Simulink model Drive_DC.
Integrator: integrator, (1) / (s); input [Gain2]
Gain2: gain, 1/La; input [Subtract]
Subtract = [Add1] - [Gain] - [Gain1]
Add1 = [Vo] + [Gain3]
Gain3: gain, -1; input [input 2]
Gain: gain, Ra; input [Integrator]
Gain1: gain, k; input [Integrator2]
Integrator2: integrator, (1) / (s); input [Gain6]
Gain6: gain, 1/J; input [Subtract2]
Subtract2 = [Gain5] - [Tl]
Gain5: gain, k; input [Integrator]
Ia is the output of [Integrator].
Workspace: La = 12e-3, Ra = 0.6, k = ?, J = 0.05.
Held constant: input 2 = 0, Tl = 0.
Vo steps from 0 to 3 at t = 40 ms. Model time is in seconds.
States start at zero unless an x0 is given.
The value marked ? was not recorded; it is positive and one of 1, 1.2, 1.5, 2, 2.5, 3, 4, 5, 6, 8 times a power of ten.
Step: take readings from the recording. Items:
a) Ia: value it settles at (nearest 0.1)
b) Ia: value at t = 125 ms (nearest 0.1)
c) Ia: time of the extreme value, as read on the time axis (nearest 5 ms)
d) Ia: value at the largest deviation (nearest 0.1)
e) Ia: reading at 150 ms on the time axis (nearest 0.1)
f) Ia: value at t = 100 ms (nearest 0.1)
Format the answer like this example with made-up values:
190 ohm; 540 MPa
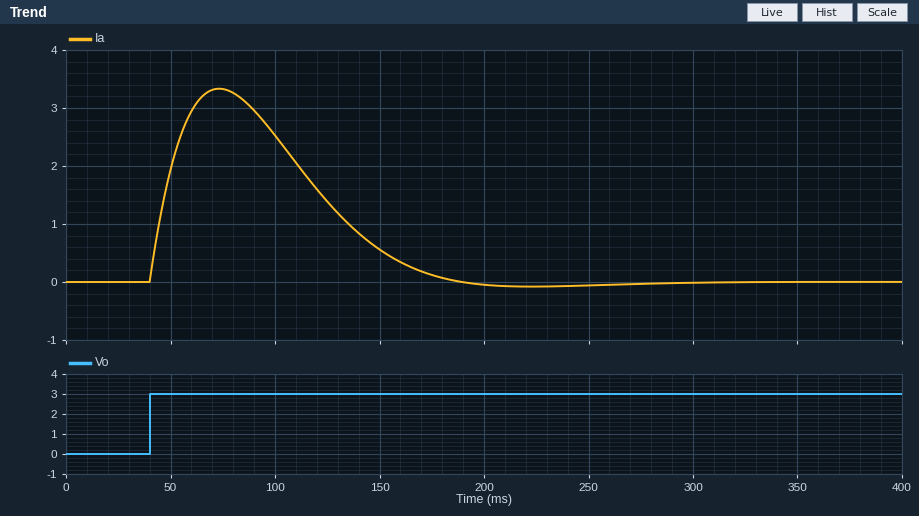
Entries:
0.0; 1.4; 75 ms; 3.3; 0.6; 2.5
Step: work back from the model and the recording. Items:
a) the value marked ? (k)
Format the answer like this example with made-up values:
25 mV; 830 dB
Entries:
0.8
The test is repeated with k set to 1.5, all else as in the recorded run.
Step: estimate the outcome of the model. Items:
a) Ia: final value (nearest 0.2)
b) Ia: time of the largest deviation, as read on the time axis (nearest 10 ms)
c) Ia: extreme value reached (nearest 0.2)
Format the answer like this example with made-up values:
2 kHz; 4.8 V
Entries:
0.0; 60 ms; 2.4
